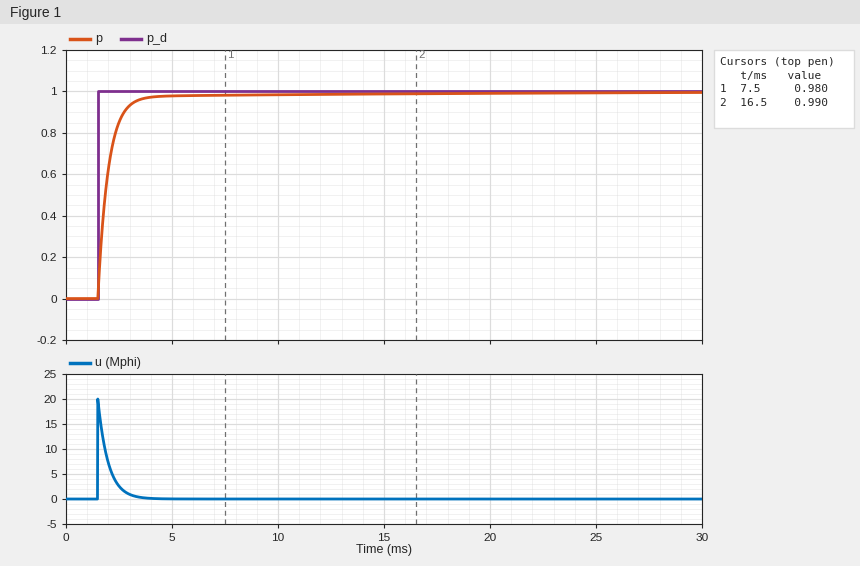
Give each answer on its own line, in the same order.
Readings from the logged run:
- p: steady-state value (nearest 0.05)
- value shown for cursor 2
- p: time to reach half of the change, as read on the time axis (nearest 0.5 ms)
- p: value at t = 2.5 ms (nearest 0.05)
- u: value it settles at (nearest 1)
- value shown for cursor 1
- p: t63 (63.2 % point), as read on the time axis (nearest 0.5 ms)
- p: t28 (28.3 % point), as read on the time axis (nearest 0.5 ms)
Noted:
1.00
0.990
2.0 ms
0.85
0
0.980
2.0 ms
1.5 ms
